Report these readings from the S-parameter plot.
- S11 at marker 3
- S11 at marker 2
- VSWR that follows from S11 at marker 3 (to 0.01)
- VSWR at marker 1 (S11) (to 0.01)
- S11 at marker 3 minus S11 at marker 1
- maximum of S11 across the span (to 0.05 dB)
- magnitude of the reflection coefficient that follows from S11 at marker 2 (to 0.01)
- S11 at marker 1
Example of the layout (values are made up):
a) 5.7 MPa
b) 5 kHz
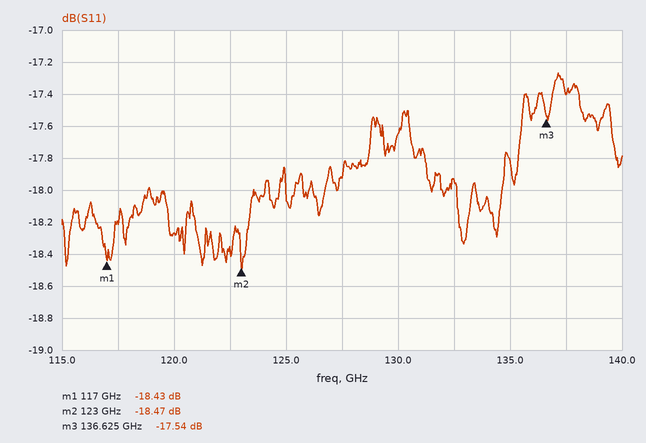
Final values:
a) -17.54 dB
b) -18.47 dB
c) 1.31
d) 1.27
e) 0.89 dB
f) -17.25 dB
g) 0.12
h) -18.43 dB
